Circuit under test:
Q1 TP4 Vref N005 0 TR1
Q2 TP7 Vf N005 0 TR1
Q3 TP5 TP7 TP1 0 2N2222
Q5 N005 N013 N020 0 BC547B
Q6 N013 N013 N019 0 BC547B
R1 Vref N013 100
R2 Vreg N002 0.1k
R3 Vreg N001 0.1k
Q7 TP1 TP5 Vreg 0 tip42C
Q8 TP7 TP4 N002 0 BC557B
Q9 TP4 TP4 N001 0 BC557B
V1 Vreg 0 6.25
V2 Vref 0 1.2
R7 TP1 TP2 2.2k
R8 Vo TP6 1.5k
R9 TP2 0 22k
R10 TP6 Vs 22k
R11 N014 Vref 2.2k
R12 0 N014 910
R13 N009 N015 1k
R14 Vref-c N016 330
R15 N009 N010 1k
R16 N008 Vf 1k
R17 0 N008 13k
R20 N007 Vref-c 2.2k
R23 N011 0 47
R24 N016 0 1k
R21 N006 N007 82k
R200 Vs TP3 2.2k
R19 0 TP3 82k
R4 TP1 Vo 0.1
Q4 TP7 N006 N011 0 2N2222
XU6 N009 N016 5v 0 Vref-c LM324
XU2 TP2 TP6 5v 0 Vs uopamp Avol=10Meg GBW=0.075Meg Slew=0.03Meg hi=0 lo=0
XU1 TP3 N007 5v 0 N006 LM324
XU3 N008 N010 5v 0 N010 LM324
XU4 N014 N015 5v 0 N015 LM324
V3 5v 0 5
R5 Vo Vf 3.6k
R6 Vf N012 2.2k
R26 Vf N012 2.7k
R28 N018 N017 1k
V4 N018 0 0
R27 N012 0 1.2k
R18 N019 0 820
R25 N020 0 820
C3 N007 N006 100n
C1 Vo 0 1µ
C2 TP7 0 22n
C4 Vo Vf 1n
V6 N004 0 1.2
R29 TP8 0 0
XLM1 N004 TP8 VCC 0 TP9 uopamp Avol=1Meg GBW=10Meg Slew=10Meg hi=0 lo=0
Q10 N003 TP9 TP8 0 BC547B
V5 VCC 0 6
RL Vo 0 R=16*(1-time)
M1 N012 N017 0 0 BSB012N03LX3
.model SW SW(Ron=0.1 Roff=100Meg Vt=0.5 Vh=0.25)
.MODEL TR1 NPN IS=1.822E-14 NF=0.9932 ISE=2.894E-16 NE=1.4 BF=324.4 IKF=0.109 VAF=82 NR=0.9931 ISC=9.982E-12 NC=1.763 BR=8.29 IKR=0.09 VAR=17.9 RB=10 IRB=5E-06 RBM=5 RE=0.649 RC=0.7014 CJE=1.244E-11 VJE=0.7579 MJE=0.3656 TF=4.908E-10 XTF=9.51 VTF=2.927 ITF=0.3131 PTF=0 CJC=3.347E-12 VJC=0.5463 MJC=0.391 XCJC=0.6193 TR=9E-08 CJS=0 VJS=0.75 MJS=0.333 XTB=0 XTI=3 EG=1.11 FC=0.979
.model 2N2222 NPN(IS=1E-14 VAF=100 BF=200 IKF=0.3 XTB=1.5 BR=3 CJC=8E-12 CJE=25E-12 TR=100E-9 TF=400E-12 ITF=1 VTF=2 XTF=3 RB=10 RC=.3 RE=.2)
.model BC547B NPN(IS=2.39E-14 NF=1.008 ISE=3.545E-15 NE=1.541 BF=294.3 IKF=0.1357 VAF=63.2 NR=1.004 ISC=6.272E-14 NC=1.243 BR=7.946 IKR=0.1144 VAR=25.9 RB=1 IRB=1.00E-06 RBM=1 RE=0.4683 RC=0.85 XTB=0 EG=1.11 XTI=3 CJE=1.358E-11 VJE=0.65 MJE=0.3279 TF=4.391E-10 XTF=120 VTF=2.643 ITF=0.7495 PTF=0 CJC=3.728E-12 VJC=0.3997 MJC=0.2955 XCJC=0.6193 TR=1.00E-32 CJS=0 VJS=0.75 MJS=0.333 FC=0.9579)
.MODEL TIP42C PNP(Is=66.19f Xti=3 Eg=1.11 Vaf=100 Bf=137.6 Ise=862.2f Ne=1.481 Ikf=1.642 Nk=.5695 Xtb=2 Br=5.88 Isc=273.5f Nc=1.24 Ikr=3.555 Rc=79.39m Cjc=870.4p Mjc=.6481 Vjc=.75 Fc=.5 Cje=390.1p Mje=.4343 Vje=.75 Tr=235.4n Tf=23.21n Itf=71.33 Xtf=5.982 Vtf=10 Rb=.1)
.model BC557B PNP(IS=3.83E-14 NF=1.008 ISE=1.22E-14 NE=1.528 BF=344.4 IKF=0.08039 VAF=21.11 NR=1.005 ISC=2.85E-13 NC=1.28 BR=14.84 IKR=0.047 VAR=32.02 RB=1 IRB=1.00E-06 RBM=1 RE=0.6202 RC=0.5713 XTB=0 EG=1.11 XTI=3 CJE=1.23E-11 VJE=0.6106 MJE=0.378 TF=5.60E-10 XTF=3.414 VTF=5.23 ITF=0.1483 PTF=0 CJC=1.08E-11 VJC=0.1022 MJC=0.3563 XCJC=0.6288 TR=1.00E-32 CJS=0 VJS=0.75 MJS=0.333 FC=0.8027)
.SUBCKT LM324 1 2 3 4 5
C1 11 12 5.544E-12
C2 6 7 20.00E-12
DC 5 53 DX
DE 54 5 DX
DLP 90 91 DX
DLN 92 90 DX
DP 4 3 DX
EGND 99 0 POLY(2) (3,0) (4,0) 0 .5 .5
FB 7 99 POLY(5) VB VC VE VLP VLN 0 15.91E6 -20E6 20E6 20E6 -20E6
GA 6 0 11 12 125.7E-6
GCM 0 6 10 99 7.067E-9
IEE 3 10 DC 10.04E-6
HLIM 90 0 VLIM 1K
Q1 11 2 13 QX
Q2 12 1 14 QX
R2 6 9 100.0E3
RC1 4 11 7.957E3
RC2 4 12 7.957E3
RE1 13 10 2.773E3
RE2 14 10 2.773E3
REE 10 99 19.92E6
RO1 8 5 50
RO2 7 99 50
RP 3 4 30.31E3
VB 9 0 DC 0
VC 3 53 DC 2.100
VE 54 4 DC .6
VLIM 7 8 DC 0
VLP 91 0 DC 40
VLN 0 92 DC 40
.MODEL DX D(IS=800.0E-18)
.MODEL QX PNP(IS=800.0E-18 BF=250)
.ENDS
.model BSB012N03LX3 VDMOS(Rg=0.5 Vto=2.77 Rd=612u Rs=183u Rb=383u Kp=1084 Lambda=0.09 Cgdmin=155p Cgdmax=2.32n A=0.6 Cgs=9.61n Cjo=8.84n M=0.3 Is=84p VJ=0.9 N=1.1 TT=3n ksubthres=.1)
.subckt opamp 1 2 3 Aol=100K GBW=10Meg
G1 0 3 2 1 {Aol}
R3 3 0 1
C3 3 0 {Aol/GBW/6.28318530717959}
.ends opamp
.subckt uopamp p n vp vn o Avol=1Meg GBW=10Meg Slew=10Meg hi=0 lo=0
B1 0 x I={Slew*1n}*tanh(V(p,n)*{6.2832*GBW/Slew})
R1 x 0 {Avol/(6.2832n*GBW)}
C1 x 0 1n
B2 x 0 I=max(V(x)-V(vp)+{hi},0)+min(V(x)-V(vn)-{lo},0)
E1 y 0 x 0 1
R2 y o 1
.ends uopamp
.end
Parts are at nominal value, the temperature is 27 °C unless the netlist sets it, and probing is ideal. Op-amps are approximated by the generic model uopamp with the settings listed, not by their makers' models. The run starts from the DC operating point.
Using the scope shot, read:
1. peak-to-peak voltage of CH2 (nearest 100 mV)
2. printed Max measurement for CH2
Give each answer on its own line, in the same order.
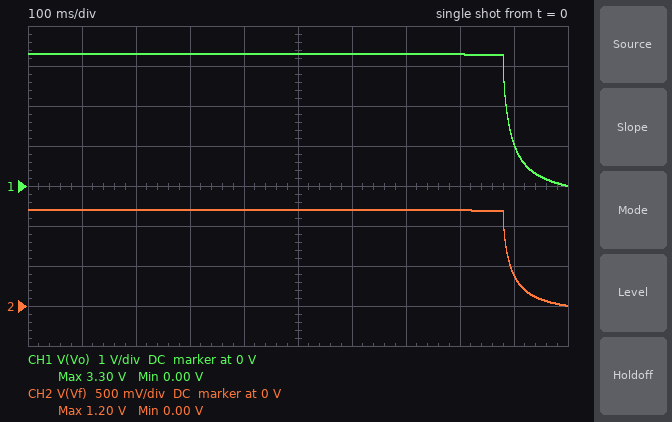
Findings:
1.2 V
1.20 V
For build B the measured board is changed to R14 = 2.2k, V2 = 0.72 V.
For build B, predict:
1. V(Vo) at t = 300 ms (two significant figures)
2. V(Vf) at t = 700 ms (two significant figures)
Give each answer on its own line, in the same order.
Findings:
2.0 V
720 mV
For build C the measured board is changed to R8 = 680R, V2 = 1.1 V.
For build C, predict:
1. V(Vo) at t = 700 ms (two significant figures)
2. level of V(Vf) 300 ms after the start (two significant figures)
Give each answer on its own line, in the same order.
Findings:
3.0 V
1.1 V
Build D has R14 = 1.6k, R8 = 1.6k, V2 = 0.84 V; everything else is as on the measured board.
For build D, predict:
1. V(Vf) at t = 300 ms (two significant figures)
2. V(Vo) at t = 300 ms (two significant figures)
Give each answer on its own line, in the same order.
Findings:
840 mV
2.3 V
